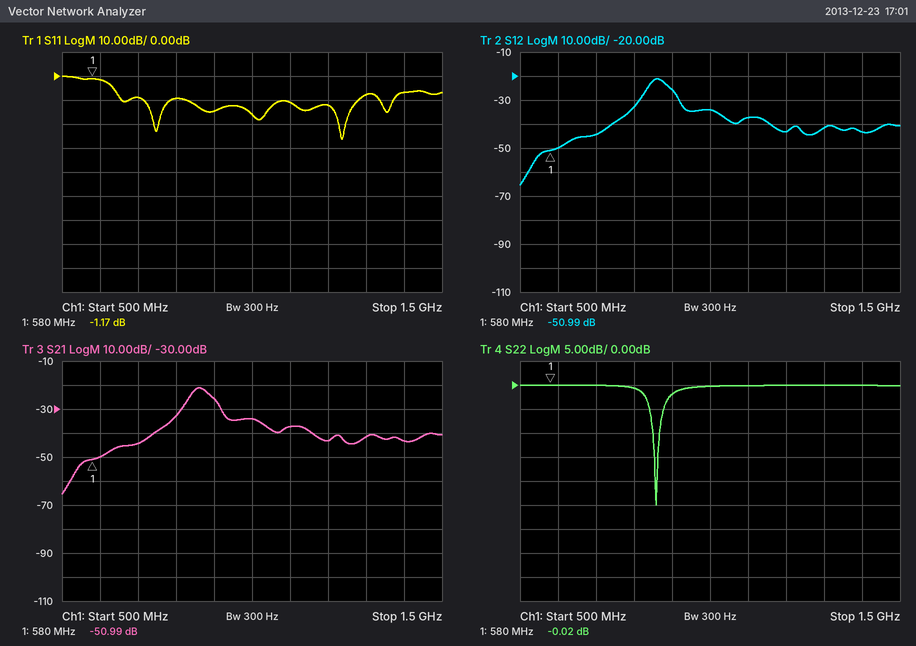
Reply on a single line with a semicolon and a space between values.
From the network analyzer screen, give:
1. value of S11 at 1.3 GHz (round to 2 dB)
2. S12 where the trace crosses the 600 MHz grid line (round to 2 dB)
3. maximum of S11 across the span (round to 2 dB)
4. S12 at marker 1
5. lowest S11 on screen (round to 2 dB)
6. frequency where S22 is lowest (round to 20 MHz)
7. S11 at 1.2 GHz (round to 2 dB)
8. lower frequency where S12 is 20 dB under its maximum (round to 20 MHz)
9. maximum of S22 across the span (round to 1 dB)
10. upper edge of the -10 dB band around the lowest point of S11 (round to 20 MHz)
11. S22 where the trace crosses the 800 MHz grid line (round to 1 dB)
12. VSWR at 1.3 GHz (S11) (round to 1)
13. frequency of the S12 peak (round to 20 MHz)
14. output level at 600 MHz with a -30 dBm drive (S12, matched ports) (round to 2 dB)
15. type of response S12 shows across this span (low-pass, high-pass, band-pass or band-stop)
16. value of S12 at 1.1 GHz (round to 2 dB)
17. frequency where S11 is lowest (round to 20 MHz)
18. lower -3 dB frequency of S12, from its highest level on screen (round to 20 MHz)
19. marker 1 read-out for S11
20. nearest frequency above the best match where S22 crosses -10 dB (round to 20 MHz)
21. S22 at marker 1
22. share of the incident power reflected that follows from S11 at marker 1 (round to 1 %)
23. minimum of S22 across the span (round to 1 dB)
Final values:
-8 dB; -50 dB; 0 dB; -50.99 dB; -26 dB; 860 MHz; -12 dB; 740 MHz; 0 dB; 1.28 GHz; -1 dB; 2; 860 MHz; -80 dBm; band-pass; -38 dB; 1.24 GHz; 840 MHz; -1.17 dB; 860 MHz; -0.02 dB; 76 %; -25 dB
